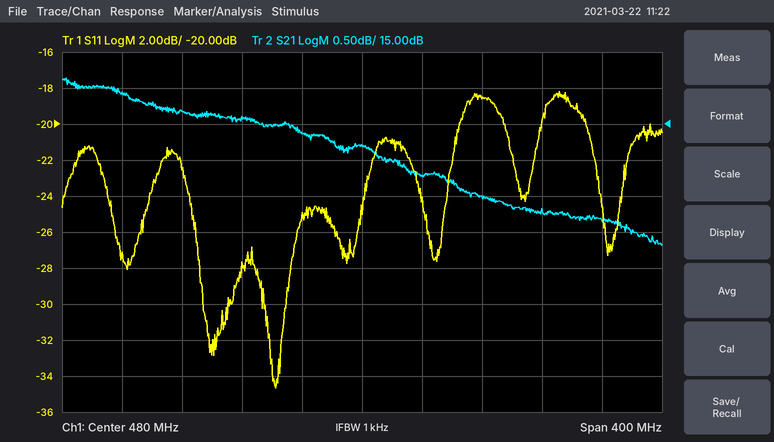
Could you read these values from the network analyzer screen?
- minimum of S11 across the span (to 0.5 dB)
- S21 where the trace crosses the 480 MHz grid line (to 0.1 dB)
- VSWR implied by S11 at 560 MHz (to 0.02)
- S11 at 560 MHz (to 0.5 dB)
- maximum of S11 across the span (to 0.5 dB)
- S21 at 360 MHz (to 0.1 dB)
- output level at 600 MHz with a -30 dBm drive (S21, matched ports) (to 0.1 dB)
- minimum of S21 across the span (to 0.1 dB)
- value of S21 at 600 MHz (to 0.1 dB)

-34.5 dB
14.7 dB
1.26
-18.5 dB
-18.0 dB
15.2 dB
-16.2 dBm
13.3 dB
13.8 dB
